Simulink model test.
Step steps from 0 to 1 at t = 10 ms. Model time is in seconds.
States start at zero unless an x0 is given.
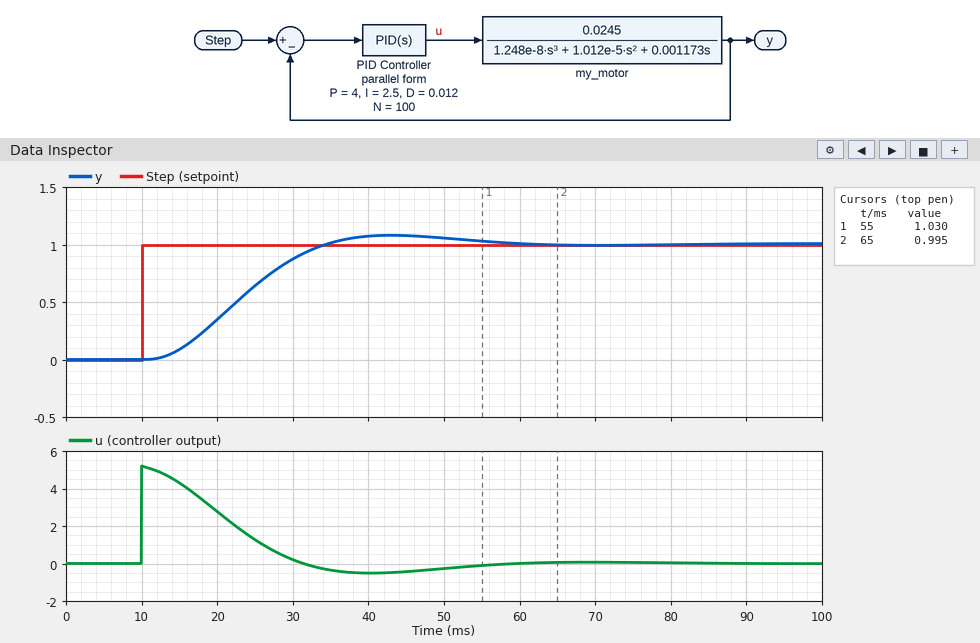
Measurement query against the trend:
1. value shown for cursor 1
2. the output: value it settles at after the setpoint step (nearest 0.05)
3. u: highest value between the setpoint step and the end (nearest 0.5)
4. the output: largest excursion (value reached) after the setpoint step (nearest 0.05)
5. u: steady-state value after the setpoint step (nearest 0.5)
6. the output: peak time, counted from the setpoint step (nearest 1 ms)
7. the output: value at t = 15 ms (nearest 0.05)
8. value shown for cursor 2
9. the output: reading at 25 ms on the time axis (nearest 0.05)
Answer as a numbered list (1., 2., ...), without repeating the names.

1. 1.030
2. 1.00
3. 5.0
4. 1.10
5. 0.0
6. 33 ms
7. 0.10
8. 0.995
9. 0.65
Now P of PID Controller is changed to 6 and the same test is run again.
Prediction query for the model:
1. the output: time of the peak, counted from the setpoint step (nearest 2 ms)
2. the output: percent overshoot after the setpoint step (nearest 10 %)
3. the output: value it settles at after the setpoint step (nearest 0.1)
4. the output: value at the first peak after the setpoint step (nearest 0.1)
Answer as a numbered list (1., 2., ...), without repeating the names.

1. 26 ms
2. 20 %
3. 1.0
4. 1.2
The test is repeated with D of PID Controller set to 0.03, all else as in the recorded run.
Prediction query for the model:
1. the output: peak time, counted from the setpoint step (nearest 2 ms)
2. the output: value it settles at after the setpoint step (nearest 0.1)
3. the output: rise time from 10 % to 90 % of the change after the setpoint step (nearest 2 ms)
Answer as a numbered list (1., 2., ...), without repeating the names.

1. 28 ms
2. 1.0
3. 14 ms
